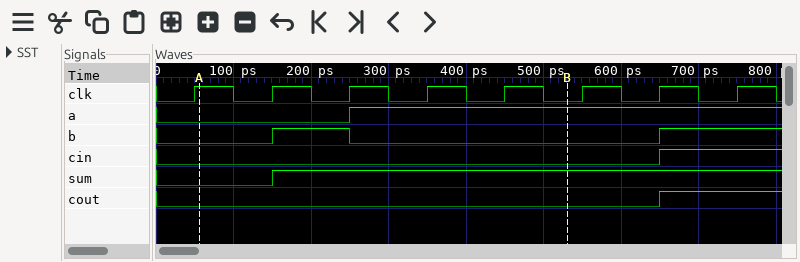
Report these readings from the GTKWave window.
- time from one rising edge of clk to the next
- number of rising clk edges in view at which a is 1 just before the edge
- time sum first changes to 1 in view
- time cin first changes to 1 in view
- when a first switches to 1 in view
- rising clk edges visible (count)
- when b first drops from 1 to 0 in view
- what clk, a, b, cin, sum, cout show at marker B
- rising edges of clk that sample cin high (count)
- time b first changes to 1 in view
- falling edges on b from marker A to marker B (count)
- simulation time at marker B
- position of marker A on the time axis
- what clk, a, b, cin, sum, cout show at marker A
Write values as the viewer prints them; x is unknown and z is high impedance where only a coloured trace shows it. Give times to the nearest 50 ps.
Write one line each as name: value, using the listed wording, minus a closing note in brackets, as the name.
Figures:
time from one rising edge of clk to the next: 100 ps
number of rising clk edges in view at which a is 1 just before the edge: 5
time sum first changes to 1 in view: 150 ps
time cin first changes to 1 in view: 650 ps
when a first switches to 1 in view: 250 ps
rising clk edges visible: 8
when b first drops from 1 to 0 in view: 250 ps
what clk, a, b, cin, sum, cout show at marker B: clk=0, a=1, b=0, cin=0, sum=1, cout=0
rising edges of clk that sample cin high: 1
time b first changes to 1 in view: 150 ps
falling edges on b from marker A to marker B: 1
simulation time at marker B: 550 ps
position of marker A on the time axis: 50 ps
what clk, a, b, cin, sum, cout show at marker A: clk=1, a=0, b=0, cin=0, sum=0, cout=0
